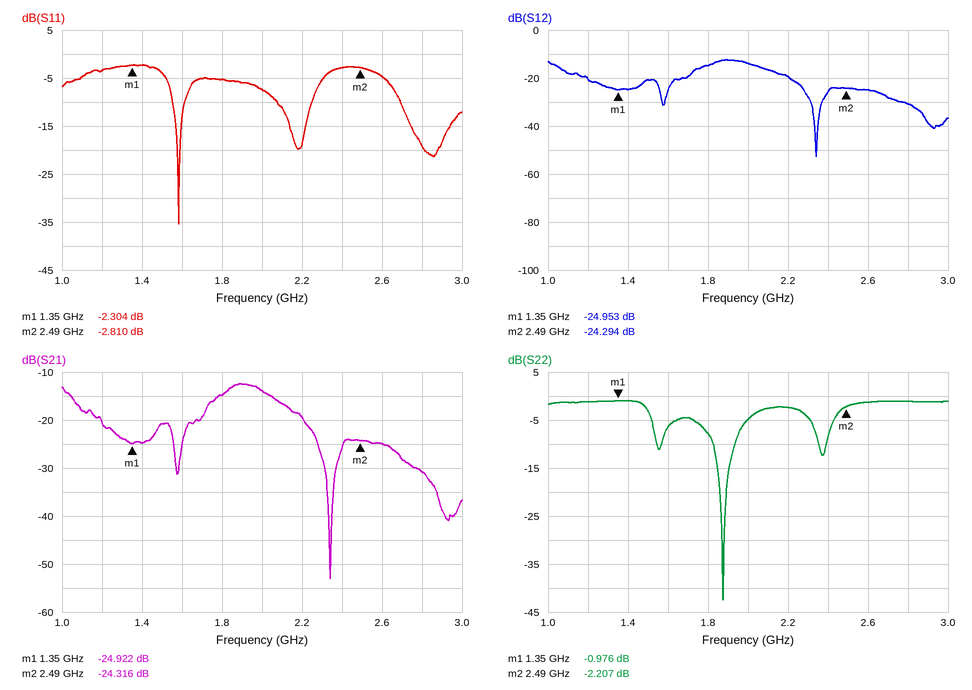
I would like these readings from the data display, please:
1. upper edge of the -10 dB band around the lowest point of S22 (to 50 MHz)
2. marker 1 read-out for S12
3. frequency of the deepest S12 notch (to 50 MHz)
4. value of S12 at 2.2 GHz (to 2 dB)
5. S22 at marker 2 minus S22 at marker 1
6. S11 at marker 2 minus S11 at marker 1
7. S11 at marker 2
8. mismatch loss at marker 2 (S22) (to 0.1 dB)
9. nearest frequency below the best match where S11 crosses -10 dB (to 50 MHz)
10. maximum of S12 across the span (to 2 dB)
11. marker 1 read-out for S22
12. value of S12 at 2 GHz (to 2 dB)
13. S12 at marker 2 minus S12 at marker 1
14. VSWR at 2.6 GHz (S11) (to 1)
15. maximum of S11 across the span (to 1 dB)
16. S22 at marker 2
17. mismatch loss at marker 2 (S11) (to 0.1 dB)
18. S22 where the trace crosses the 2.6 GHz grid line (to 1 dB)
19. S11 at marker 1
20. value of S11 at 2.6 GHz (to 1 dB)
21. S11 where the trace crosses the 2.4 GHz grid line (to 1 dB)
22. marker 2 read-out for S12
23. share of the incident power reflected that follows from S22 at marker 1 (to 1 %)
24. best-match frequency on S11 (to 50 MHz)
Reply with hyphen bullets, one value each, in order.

- 1.95 GHz
- -24.953 dB
- 2.35 GHz
- -20 dB
- -1.231 dB
- -0.506 dB
- -2.810 dB
- 4.0 dB
- 1.55 GHz
- -12 dB
- -0.976 dB
- -14 dB
- 0.659 dB
- 4
- -2 dB
- -2.207 dB
- 3.2 dB
- -1 dB
- -2.304 dB
- -5 dB
- -3 dB
- -24.294 dB
- 80 %
- 1.60 GHz
